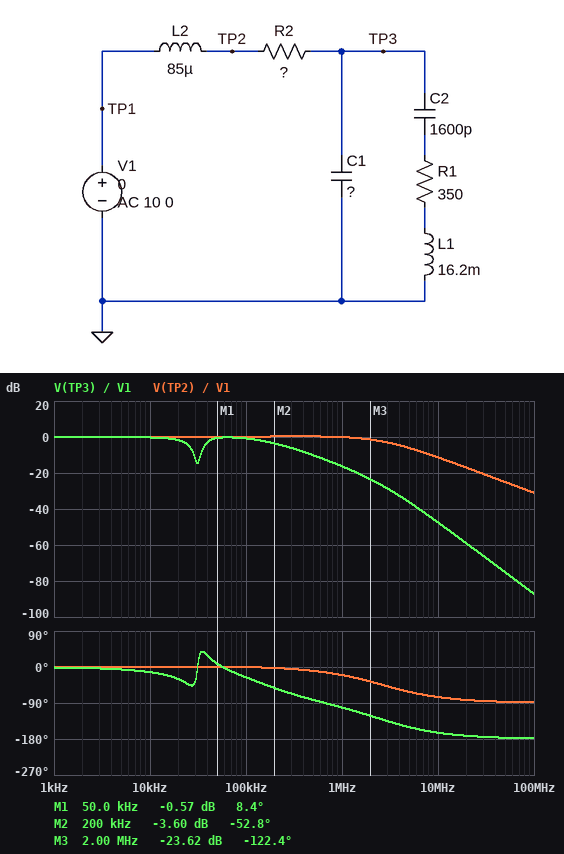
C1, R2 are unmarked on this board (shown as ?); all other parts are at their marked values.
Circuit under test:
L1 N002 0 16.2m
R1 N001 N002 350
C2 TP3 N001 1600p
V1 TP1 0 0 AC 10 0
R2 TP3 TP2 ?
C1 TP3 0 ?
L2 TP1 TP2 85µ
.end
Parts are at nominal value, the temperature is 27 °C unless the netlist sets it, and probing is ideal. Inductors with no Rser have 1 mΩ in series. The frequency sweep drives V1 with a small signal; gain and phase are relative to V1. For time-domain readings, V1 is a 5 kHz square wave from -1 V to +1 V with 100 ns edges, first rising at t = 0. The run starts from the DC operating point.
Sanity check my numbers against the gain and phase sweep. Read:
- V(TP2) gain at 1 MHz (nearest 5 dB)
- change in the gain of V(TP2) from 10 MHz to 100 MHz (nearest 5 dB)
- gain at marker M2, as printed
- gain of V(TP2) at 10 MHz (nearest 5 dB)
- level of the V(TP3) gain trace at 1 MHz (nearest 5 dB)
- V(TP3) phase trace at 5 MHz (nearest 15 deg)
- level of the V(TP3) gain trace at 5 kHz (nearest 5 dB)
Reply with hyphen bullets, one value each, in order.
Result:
- 0 dB
- -20 dB
- -3.60 dB
- -10 dB
- -15 dB
- -150 deg
- 0 dB
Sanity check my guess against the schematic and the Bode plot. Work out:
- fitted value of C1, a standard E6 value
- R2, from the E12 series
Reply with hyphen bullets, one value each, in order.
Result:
- 680 pF
- 1.5 kΩ
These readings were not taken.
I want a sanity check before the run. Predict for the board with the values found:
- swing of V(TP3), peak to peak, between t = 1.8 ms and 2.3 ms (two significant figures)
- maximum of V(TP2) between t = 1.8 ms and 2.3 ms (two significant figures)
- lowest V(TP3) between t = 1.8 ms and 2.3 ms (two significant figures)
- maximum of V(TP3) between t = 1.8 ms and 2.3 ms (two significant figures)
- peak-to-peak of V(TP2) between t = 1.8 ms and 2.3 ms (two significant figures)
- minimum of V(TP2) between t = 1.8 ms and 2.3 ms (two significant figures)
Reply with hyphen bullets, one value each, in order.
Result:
- 2.5 V
- 1.1 V
- -1.2 V
- 1.2 V
- 2.2 V
- -1.1 V
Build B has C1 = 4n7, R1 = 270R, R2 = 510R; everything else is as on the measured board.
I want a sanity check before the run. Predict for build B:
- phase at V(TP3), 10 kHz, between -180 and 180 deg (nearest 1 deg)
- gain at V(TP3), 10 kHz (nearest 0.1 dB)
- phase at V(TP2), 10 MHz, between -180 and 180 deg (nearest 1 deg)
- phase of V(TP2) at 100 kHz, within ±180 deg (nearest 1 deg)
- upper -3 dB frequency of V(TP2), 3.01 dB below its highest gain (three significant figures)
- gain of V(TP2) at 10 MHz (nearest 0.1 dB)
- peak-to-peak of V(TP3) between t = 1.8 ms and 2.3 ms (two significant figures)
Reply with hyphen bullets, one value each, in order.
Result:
- -12 deg
- -0.2 dB
- -85 deg
- -4 deg
- 930 kHz
- -20.4 dB
- 2.3 V
